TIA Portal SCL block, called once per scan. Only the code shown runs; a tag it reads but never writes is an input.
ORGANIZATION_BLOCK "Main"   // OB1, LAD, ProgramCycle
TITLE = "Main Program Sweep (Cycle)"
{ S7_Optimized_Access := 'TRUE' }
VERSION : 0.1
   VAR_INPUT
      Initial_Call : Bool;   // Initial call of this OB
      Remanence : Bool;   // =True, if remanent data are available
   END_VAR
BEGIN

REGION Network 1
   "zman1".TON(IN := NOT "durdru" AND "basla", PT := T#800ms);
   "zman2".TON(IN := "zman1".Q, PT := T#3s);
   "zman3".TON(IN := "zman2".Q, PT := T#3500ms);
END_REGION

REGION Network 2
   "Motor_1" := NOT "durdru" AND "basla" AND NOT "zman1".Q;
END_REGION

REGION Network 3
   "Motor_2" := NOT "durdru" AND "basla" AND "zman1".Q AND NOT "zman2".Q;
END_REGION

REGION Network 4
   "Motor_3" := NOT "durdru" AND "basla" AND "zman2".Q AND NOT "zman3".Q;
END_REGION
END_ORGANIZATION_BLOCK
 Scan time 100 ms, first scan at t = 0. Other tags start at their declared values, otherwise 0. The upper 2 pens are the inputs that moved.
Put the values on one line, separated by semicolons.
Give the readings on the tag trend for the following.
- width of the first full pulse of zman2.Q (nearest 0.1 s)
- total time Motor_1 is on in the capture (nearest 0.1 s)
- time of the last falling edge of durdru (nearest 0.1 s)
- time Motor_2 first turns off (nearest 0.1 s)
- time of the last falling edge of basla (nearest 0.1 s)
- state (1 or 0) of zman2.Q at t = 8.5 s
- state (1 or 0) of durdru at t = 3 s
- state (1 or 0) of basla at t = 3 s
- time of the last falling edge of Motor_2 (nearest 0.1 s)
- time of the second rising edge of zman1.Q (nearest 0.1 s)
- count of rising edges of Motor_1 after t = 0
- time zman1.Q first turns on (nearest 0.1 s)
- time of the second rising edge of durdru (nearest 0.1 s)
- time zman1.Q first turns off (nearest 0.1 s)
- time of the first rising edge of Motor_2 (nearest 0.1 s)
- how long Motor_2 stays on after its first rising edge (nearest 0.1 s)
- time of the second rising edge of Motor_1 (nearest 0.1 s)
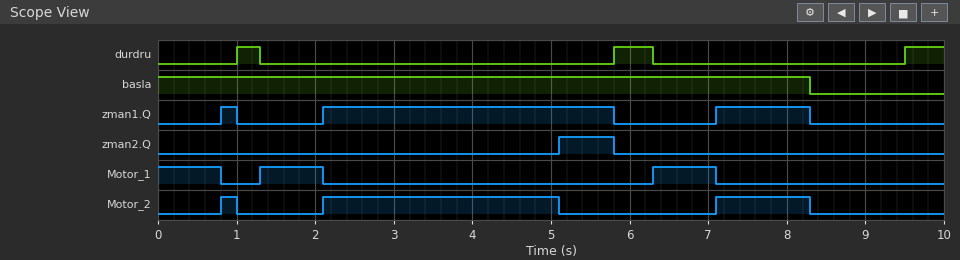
0.7 s; 2.4 s; 6.3 s; 1.0 s; 8.3 s; 0; 0; 1; 8.3 s; 2.1 s; 2; 0.8 s; 5.8 s; 1.0 s; 0.8 s; 0.2 s; 6.3 s
